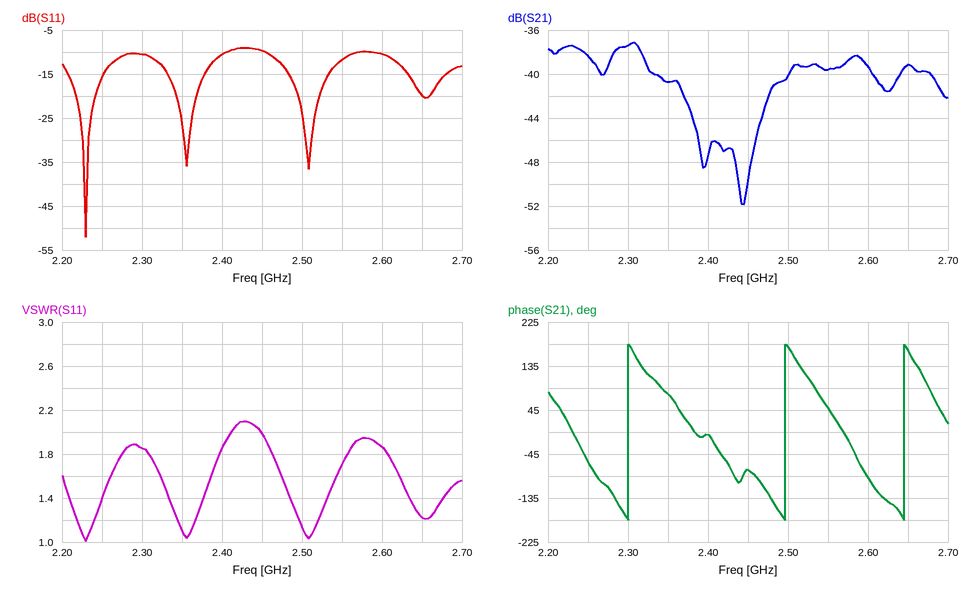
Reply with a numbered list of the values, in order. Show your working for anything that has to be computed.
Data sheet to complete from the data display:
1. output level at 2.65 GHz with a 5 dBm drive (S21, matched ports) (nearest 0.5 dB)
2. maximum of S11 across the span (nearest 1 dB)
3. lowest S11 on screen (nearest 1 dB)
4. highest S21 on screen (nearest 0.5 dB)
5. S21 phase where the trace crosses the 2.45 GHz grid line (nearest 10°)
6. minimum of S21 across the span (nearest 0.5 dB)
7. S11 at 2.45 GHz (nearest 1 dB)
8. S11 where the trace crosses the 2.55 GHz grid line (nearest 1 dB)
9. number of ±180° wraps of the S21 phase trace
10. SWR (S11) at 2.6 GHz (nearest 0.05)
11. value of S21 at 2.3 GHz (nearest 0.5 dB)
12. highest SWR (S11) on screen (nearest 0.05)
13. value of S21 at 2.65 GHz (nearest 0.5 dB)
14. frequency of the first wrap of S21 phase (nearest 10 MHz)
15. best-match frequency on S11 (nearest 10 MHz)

1. 5 dBm + (-39.0 dB) = -34.0 dBm
2. -9 dB
3. -52 dB
4. -37.0 dB
5. -80°
6. -52.0 dB
7. -10 dB
8. -12 dB
9. 3
10. 1.85
11. -37.5 dB
12. 2.10
13. -39.0 dB
14. 2.30 GHz
15. 2.23 GHz
